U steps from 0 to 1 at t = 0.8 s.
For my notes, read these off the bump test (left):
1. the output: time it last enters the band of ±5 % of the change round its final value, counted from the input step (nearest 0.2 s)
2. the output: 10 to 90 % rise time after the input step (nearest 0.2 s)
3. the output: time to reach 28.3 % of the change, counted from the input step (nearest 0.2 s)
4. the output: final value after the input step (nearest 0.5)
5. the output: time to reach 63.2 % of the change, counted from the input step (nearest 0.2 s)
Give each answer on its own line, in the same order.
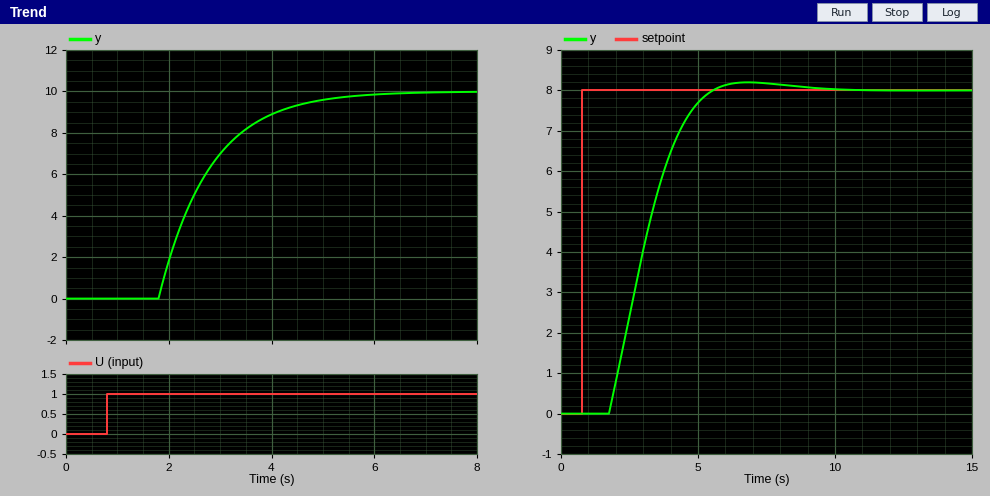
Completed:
4.0 s
2.2 s
1.4 s
10.0
2.0 s
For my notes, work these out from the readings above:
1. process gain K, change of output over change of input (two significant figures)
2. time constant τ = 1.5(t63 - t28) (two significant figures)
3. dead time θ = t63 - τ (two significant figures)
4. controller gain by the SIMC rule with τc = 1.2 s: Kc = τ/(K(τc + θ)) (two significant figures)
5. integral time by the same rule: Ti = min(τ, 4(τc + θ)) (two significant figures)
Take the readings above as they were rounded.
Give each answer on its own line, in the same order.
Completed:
10
0.90 s
1.1 s
0.039
0.90 s
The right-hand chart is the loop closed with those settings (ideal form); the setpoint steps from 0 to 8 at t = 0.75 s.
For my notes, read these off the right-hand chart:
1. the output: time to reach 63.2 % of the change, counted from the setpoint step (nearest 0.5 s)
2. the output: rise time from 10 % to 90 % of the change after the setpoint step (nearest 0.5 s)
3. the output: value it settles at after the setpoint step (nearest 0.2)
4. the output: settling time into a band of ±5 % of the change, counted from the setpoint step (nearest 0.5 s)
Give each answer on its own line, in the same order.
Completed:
2.5 s
2.5 s
8.0
4.0 s
